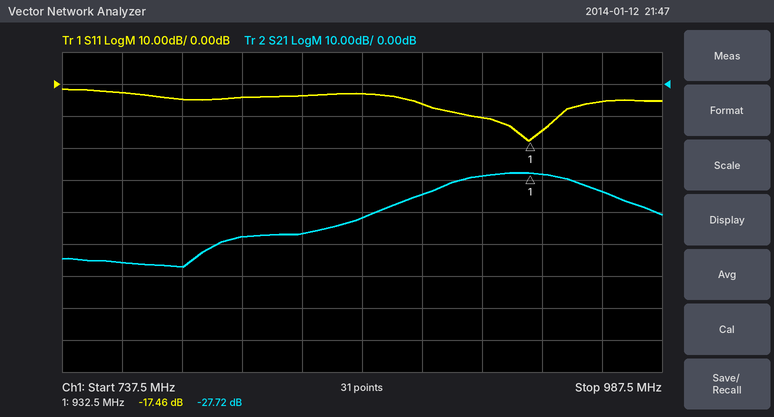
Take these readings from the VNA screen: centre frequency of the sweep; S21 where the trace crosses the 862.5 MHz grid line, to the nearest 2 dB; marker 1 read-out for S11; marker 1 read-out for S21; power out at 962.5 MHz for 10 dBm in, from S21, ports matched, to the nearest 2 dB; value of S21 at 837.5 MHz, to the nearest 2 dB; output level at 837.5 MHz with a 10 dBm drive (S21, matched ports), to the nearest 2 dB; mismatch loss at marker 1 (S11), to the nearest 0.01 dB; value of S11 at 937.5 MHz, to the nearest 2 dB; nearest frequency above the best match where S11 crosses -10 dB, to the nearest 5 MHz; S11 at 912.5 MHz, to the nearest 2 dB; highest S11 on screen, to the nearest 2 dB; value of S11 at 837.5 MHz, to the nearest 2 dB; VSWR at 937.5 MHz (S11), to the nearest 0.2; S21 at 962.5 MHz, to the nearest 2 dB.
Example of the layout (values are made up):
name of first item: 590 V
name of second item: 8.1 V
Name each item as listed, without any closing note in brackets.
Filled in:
centre frequency of the sweep: 862.5 MHz
S21 where the trace crosses the 862.5 MHz grid line, to the nearest 2 dB: -42 dB
marker 1 read-out for S11: -17.46 dB
marker 1 read-out for S21: -27.72 dB
power out at 962.5 MHz for 10 dBm in, from S21, ports matched, to the nearest 2 dB: -24 dBm
value of S21 at 837.5 MHz, to the nearest 2 dB: -46 dB
output level at 837.5 MHz with a 10 dBm drive (S21, matched ports), to the nearest 2 dB: -36 dBm
mismatch loss at marker 1 (S11), to the nearest 0.01 dB: 0.08 dB
value of S11 at 937.5 MHz, to the nearest 2 dB: -14 dB
nearest frequency above the best match where S11 crosses -10 dB, to the nearest 5 MHz: 945 MHz
S11 at 912.5 MHz, to the nearest 2 dB: -10 dB
highest S11 on screen, to the nearest 2 dB: -2 dB
value of S11 at 837.5 MHz, to the nearest 2 dB: -4 dB
VSWR at 937.5 MHz (S11), to the nearest 0.2: 1.4
S21 at 962.5 MHz, to the nearest 2 dB: -34 dB
